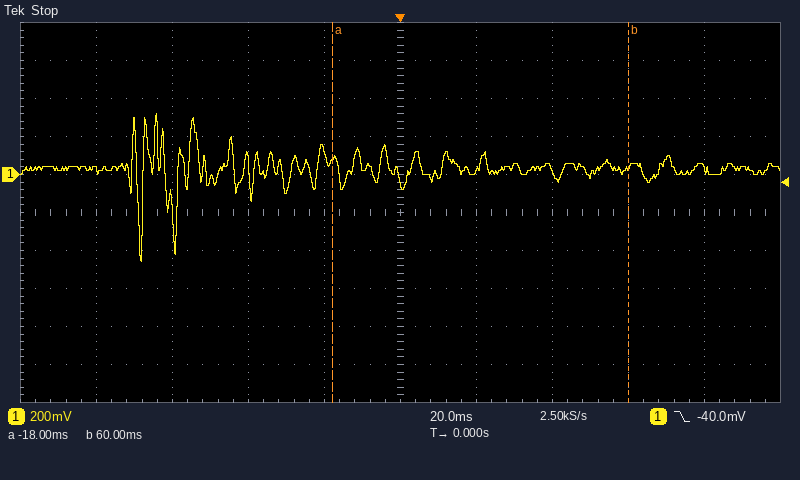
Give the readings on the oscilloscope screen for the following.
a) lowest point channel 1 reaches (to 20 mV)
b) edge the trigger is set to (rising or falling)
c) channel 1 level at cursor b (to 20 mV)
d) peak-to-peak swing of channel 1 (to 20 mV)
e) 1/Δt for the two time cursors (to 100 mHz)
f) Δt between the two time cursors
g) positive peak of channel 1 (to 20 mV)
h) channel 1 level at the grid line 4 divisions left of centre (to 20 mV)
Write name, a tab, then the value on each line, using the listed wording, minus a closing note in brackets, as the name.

lowest point channel 1 reaches	-460 mV
edge the trigger is set to	falling
channel 1 level at cursor b	40 mV
peak-to-peak swing of channel 1	780 mV
1/Δt for the two time cursors	12.8 Hz
Δt between the two time cursors	78 ms
positive peak of channel 1	320 mV
channel 1 level at the grid line 4 divisions left of centre	20 mV
